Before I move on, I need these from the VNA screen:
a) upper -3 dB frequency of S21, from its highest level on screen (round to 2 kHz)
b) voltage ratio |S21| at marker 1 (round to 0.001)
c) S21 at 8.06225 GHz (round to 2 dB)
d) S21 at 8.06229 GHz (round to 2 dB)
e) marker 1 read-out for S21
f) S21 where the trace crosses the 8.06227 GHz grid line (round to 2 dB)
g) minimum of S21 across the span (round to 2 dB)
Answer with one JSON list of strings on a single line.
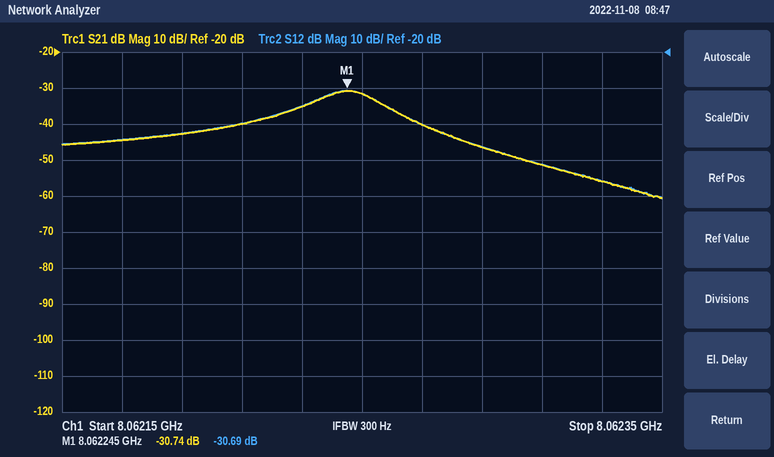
["8.062256 GHz", "0.029", "-32 dB", "-46 dB", "-30.74 dB", "-40 dB", "-60 dB"]
